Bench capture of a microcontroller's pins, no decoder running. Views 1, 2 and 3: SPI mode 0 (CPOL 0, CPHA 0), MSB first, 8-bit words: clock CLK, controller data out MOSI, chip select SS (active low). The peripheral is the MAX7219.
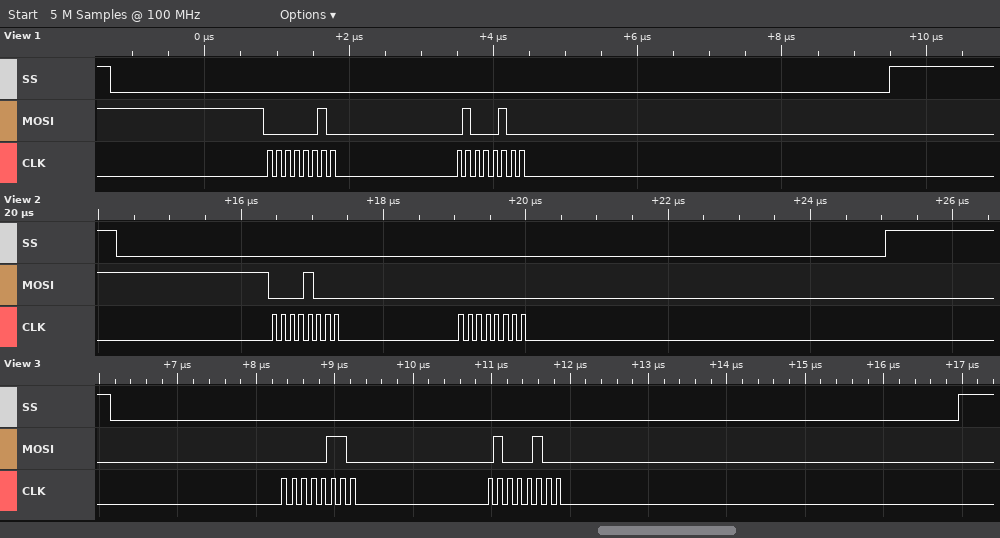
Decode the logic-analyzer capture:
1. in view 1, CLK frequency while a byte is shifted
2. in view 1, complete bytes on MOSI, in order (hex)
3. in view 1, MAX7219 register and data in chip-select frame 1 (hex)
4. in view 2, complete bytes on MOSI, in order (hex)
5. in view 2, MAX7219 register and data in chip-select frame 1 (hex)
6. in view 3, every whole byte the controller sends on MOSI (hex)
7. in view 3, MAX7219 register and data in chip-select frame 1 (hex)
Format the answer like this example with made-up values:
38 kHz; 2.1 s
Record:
8 MHz; 0x02 0x44; register 0x2, data 0x44; 08 00; register 0x8, data 0x00; 06 44; register 0x6, data 0x44
